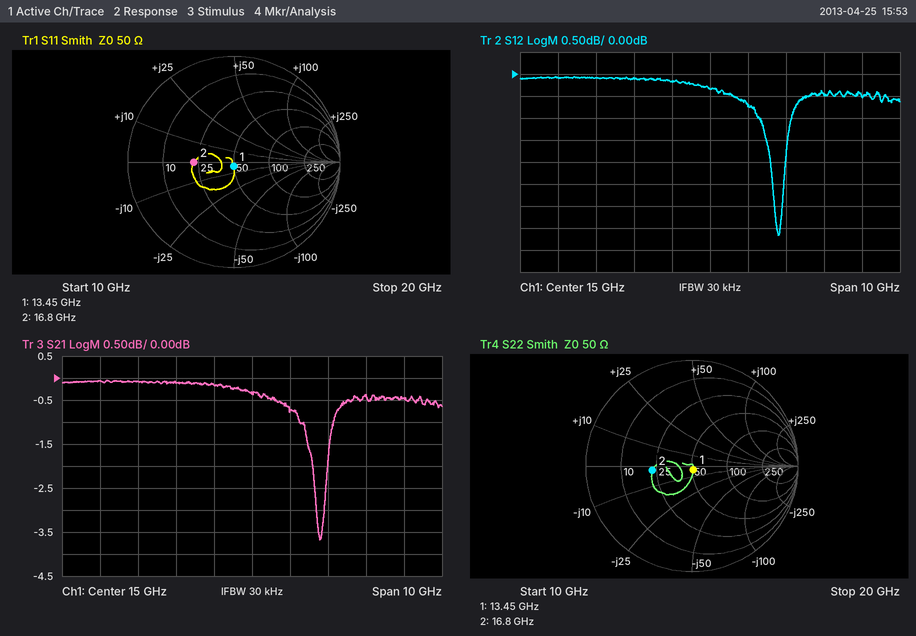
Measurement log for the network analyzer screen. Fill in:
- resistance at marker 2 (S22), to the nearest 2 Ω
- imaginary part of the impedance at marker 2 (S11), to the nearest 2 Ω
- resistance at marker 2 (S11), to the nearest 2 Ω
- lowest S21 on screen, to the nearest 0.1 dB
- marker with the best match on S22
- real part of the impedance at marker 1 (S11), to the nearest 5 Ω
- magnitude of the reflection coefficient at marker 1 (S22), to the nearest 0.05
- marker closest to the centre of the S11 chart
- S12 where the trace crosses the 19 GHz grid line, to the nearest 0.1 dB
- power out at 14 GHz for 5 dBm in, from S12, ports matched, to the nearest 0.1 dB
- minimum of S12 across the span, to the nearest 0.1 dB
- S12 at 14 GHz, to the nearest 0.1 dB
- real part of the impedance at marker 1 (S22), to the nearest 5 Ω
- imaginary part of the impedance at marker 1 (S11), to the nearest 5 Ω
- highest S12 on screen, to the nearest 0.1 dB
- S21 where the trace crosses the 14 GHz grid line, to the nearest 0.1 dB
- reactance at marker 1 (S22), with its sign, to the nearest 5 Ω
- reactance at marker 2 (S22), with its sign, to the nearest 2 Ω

22 Ω
0 Ω
22 Ω
-3.7 dB
marker 1
50 Ω
0.05
marker 1
-0.5 dB
4.8 dBm
-3.7 dB
-0.2 dB
50 Ω
-5 Ω
-0.1 dB
-0.2 dB
-5 Ω
-2 Ω
